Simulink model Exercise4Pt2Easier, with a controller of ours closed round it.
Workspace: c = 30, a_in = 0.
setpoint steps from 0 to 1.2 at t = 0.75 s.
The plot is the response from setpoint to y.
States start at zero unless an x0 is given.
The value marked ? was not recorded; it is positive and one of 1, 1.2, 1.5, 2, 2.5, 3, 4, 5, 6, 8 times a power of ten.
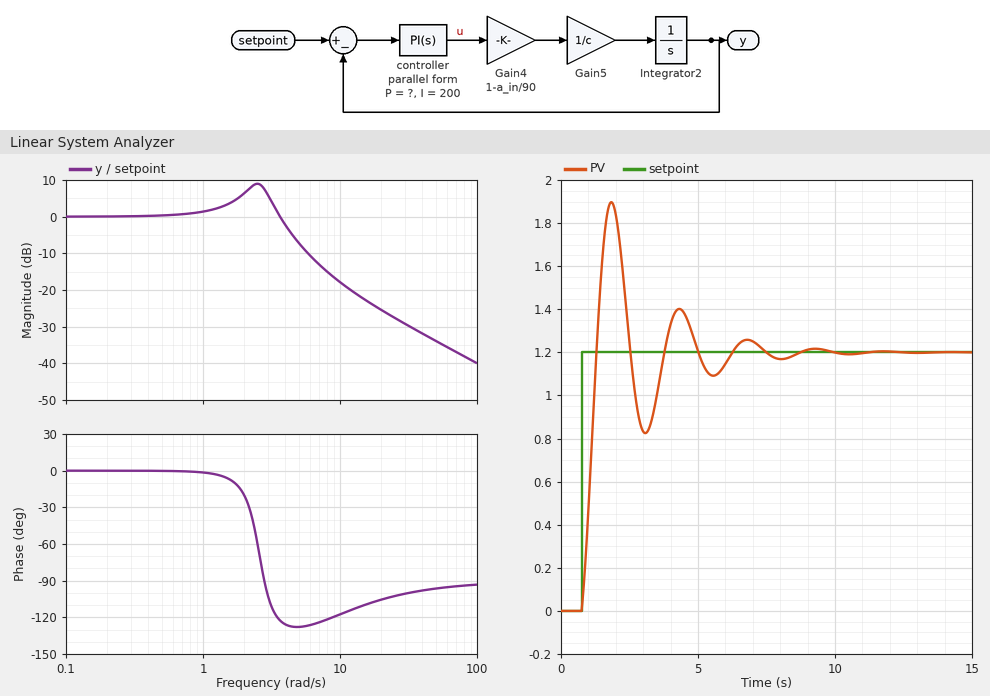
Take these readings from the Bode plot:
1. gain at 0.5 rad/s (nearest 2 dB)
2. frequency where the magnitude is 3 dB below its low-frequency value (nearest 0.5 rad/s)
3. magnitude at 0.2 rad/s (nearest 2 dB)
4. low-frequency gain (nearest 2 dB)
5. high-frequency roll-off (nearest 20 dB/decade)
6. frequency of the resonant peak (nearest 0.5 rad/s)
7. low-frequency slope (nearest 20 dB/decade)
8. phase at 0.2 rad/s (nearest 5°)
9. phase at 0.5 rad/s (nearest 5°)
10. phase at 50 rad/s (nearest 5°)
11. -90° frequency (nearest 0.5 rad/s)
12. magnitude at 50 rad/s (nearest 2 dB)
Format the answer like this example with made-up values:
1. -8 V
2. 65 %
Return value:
1. 0 dB
2. 4.0 rad/s
3. 0 dB
4. 0 dB
5. -20 dB/decade
6. 2.5 rad/s
7. 0 dB/decade
8. 0°
9. 0°
10. -95°
11. 3.0 rad/s
12. -34 dB
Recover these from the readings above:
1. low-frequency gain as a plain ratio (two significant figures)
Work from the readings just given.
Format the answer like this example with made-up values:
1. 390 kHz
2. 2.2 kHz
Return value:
1. 1.0
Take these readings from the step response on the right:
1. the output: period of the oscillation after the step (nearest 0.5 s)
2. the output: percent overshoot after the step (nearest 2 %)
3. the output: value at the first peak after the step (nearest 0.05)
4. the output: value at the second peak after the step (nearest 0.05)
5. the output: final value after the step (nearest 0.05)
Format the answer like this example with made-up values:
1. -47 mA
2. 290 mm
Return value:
1. 2.5 s
2. 58 %
3. 1.90
4. 1.40
5. 1.20
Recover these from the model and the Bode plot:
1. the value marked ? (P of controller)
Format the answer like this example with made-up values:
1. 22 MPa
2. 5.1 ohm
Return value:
1. 30
